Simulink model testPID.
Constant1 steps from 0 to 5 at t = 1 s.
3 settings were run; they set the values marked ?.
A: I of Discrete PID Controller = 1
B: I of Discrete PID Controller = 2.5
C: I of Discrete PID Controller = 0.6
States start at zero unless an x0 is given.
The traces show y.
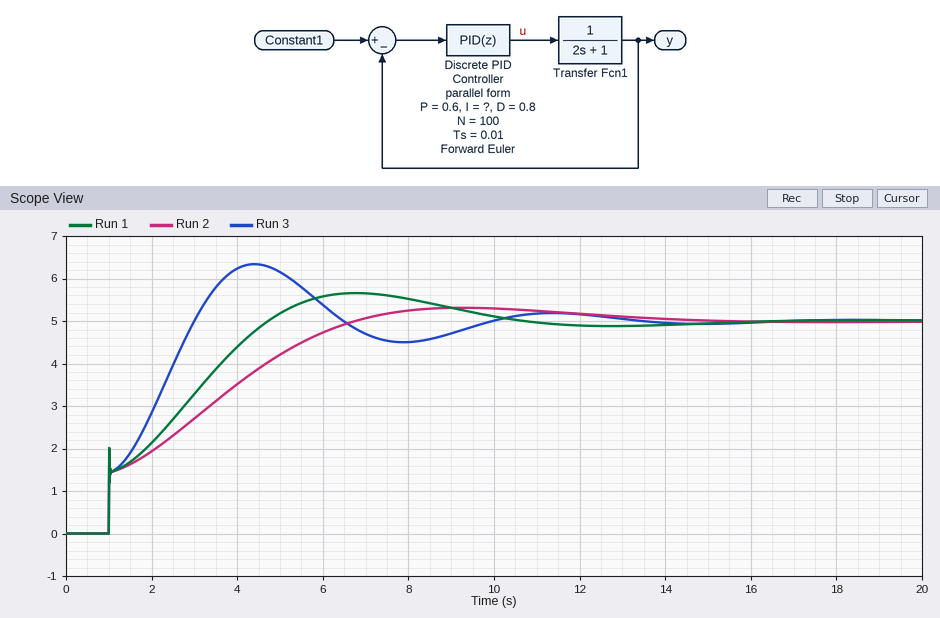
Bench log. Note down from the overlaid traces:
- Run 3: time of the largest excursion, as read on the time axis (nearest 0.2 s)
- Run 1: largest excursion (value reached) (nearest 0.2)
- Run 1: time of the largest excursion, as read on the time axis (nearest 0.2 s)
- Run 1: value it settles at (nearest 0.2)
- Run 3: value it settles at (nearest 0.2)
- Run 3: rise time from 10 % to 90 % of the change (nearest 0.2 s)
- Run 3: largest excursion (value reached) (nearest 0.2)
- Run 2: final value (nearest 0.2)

4.4 s
5.6
6.8 s
5.0
5.0
1.8 s
6.4
5.0
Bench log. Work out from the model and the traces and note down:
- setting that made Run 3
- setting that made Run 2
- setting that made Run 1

B
C
A
